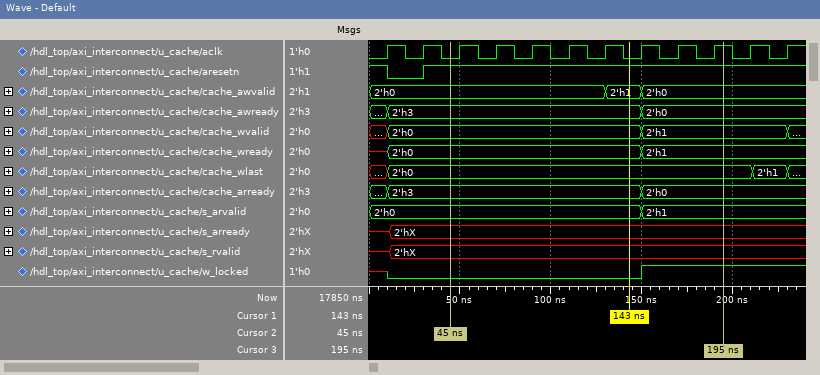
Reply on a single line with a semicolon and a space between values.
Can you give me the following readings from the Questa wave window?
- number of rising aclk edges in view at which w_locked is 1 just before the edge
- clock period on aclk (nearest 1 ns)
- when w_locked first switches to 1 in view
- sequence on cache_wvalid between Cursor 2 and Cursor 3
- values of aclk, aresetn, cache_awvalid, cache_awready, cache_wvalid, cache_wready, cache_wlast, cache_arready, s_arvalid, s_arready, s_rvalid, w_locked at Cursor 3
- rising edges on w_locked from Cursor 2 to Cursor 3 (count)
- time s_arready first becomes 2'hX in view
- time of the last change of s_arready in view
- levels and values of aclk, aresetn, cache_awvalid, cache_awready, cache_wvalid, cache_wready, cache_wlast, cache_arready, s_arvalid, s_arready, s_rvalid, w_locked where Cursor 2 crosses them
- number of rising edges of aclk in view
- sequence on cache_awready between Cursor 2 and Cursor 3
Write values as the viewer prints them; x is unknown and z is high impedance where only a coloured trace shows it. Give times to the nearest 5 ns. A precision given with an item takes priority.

4; 20 ns; 150 ns; 2'h0, 2'h1; aclk=1, aresetn=1, cache_awvalid=2'h0, cache_awready=2'h0, cache_wvalid=2'h1, cache_wready=2'h1, cache_wlast=2'h0, cache_arready=2'h0, s_arvalid=2'h1, s_arready=2'hX, s_rvalid=2'hX, w_locked=1; 1; 10 ns; 10 ns; aclk=0, aresetn=1, cache_awvalid=2'h0, cache_awready=2'h3, cache_wvalid=2'h0, cache_wready=2'h0, cache_wlast=2'h0, cache_arready=2'h3, s_arvalid=2'h0, s_arready=2'hX, s_rvalid=2'hX, w_locked=0; 12; 2'h3, 2'h0
